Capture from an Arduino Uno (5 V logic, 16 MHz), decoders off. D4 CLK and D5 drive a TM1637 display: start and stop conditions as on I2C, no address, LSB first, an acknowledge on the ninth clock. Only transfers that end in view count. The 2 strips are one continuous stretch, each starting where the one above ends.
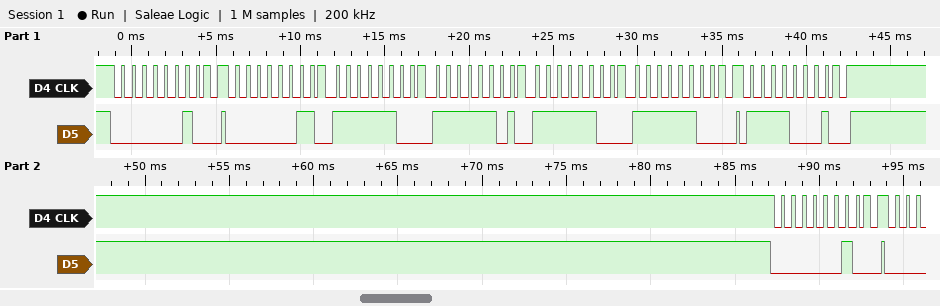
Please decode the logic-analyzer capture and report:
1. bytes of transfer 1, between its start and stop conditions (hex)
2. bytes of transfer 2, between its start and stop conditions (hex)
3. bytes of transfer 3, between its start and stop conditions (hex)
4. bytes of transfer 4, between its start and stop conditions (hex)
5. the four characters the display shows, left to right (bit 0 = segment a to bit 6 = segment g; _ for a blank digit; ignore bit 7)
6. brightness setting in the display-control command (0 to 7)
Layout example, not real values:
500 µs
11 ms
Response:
40
C0 3F BF 3F 3F
8F
40
0000
7
